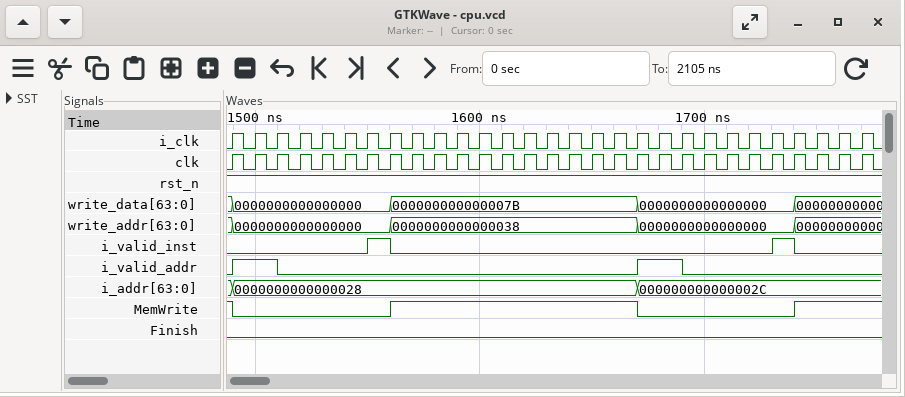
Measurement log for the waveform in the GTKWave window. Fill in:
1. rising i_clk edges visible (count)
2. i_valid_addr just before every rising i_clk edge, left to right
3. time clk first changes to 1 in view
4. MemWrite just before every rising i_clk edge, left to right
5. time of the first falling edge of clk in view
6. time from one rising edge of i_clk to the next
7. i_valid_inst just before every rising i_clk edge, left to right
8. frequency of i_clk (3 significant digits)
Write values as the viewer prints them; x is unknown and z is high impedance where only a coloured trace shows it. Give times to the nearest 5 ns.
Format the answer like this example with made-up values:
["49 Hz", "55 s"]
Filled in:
["29", "0 1 1 0 0 0 0 0 0 0 0 0 0 0 0 0 0 0 0 1 1 0 0 0 0 0 0 0 0", "1490 ns", "1 0 0 0 0 0 0 0 1 1 1 1 1 1 1 1 1 1 1 0 0 0 0 0 0 0 1 1 1", "1495 ns", "10 ns", "0 0 0 0 0 0 0 1 0 0 0 0 0 0 0 0 0 0 0 0 0 0 0 0 0 1 0 0 0", "100 MHz"]
